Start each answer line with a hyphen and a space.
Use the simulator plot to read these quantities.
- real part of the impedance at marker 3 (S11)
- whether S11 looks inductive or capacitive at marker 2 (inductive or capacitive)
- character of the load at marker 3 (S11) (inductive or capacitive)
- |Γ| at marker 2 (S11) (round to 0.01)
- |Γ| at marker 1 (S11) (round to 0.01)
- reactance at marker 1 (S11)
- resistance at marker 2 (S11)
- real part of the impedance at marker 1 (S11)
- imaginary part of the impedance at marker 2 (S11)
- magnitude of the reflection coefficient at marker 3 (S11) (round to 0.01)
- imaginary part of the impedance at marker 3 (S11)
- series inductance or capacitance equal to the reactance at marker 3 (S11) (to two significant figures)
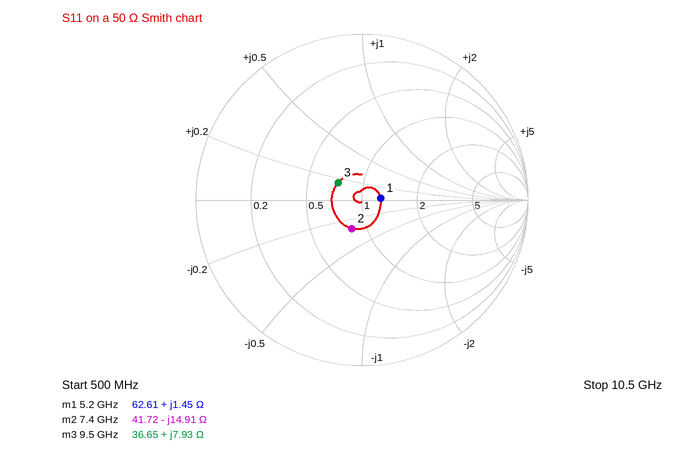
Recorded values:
- 36.65 Ω
- capacitive
- inductive
- 0.18
- 0.11
- +1.45 Ω
- 41.72 Ω
- 62.61 Ω
- -14.91 Ω
- 0.18
- +7.93 Ω
- 130 pH
